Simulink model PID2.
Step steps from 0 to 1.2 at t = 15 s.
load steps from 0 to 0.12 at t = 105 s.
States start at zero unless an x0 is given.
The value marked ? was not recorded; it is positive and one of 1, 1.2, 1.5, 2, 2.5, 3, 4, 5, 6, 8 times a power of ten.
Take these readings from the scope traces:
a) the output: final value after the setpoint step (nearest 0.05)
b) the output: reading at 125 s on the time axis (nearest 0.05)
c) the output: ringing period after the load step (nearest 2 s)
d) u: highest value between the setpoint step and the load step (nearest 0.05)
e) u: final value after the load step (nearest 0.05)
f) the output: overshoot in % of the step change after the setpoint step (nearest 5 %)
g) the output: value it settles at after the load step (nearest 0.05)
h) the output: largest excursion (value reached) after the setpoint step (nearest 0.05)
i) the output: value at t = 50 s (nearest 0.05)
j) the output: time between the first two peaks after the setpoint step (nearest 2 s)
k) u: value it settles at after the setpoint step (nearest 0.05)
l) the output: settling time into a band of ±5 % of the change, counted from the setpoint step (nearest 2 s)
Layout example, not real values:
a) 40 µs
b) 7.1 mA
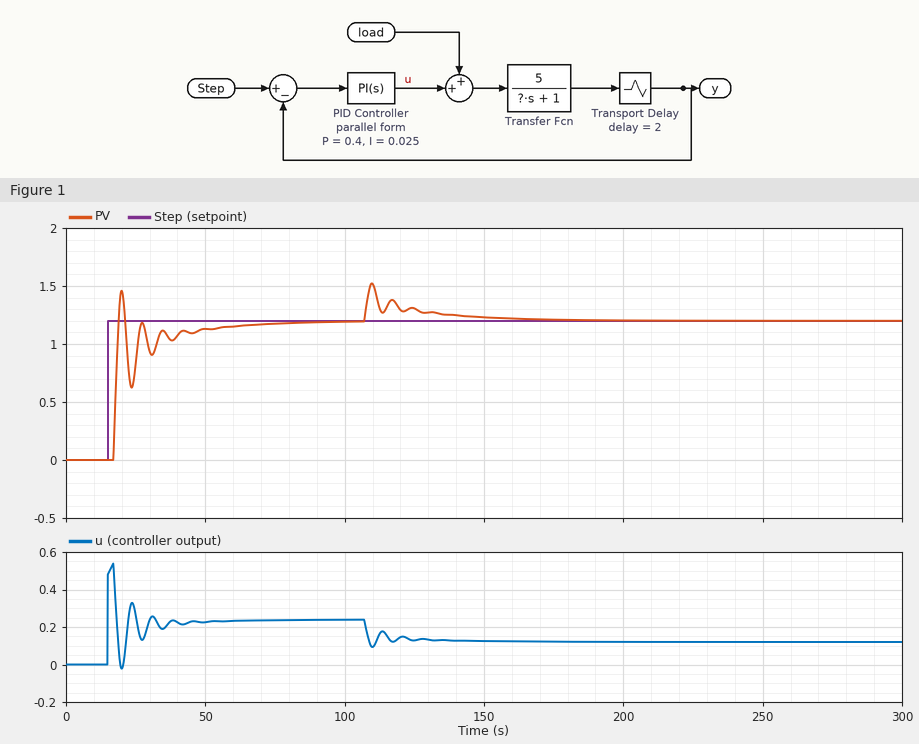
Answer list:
a) 1.20
b) 1.30
c) 8 s
d) 0.55
e) 0.10
f) 20 %
g) 1.20
h) 1.45
i) 1.15
j) 8 s
k) 0.25
l) 40 s
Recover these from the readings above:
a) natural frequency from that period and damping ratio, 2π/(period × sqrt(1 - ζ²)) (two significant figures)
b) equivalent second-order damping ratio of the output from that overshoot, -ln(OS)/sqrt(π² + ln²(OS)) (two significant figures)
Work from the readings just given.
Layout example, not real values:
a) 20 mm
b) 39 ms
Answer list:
a) 0.88 rad/s
b) 0.46
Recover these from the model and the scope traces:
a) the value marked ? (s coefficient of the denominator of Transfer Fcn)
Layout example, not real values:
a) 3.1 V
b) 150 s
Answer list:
a) 3
